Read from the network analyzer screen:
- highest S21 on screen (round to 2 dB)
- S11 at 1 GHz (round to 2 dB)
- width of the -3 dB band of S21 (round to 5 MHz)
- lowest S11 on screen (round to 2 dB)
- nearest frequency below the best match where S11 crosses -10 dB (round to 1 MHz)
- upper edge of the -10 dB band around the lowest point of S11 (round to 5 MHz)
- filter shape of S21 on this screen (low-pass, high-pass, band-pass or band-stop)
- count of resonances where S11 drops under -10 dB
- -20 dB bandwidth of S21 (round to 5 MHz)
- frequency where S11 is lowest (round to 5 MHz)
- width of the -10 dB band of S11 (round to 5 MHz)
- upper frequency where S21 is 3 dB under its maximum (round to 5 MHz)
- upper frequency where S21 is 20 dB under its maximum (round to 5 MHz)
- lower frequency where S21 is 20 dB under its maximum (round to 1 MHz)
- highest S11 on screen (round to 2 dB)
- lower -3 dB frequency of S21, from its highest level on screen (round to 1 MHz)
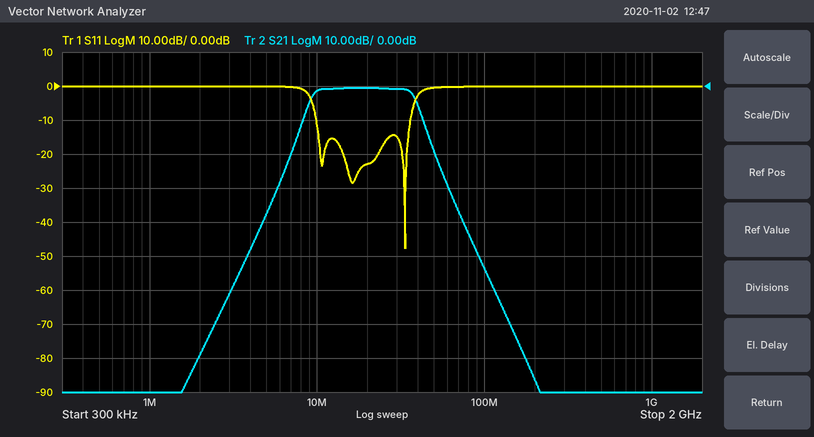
0 dB
0 dB
30 MHz
-48 dB
10 MHz
35 MHz
band-pass
3
45 MHz
35 MHz
25 MHz
40 MHz
50 MHz
7 MHz
0 dB
9 MHz
